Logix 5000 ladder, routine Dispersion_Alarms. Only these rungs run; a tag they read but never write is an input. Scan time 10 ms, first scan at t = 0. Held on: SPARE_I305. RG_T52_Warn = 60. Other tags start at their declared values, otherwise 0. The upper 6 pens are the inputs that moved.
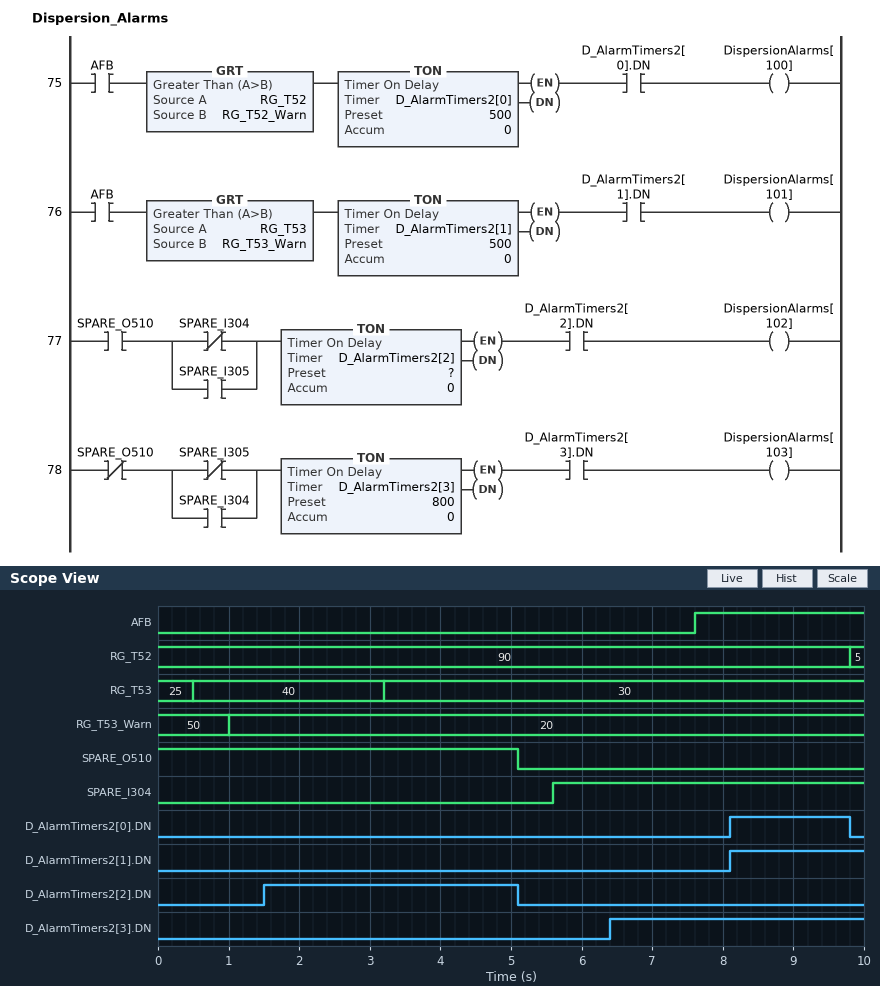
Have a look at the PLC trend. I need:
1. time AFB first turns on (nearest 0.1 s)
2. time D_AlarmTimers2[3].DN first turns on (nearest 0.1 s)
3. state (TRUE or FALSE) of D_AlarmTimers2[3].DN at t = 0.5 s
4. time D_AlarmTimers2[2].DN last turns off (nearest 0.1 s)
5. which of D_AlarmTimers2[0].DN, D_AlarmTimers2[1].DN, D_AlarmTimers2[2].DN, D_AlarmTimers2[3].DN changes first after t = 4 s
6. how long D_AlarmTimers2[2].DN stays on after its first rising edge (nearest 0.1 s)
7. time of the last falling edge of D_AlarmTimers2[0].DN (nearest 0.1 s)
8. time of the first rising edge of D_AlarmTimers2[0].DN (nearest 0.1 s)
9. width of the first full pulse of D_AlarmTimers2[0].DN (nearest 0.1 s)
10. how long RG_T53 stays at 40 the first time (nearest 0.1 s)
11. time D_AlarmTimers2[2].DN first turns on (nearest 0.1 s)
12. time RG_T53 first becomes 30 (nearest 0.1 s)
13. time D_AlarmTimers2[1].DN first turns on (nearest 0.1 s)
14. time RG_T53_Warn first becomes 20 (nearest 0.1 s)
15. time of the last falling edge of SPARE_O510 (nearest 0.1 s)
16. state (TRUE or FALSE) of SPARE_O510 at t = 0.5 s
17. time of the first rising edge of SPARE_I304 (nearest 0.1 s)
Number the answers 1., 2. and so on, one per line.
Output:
1. 7.6 s
2. 6.4 s
3. FALSE
4. 5.1 s
5. D_AlarmTimers2[2].DN
6. 3.6 s
7. 9.8 s
8. 8.1 s
9. 1.7 s
10. 2.7 s
11. 1.5 s
12. 3.2 s
13. 8.1 s
14. 1.0 s
15. 5.1 s
16. TRUE
17. 5.6 s
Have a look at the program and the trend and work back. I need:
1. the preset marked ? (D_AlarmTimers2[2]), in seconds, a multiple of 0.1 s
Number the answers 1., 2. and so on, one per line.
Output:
1. 1.5 s
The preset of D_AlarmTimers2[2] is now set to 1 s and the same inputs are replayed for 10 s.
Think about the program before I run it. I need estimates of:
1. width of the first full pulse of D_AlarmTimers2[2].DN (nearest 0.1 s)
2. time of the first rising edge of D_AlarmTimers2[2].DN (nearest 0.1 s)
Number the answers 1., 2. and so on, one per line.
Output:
1. 4.1 s
2. 1.0 s
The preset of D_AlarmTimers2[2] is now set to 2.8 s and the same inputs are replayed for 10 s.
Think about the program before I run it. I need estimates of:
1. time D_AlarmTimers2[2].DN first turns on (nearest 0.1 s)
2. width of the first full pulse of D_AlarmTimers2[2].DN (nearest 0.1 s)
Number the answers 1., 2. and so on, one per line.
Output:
1. 2.8 s
2. 2.3 s
